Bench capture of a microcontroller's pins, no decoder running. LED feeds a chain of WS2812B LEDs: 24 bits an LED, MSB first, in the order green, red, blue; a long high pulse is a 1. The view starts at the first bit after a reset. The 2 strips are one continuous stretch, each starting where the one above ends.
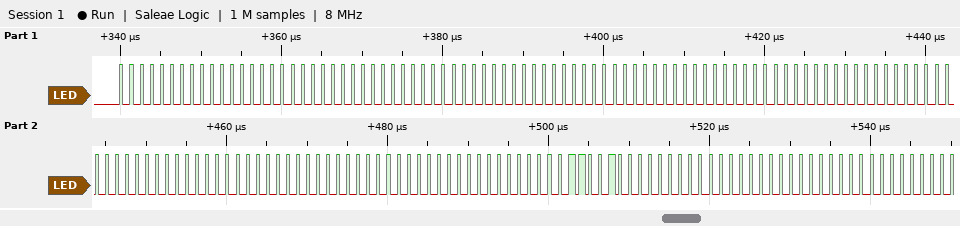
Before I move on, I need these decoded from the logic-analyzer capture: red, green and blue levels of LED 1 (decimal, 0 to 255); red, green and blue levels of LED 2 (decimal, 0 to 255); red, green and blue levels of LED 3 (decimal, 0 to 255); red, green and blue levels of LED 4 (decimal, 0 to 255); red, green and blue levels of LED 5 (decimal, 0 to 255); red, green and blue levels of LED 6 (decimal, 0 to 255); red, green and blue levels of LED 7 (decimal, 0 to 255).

0, 0, 0
0, 0, 0
0, 0, 0
0, 0, 0
0, 0, 0
50, 0, 0
0, 0, 0
